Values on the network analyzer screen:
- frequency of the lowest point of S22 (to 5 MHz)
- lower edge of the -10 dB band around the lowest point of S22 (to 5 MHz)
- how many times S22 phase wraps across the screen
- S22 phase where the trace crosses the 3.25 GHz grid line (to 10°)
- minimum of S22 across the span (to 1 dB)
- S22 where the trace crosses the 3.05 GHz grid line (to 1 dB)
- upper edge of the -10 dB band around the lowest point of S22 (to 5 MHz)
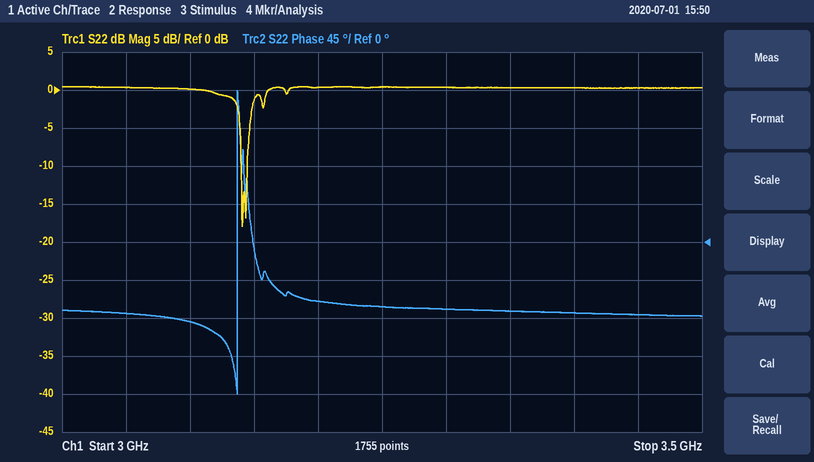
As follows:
3.140 GHz
3.140 GHz
1
-80°
-18 dB
0 dB
3.145 GHz
